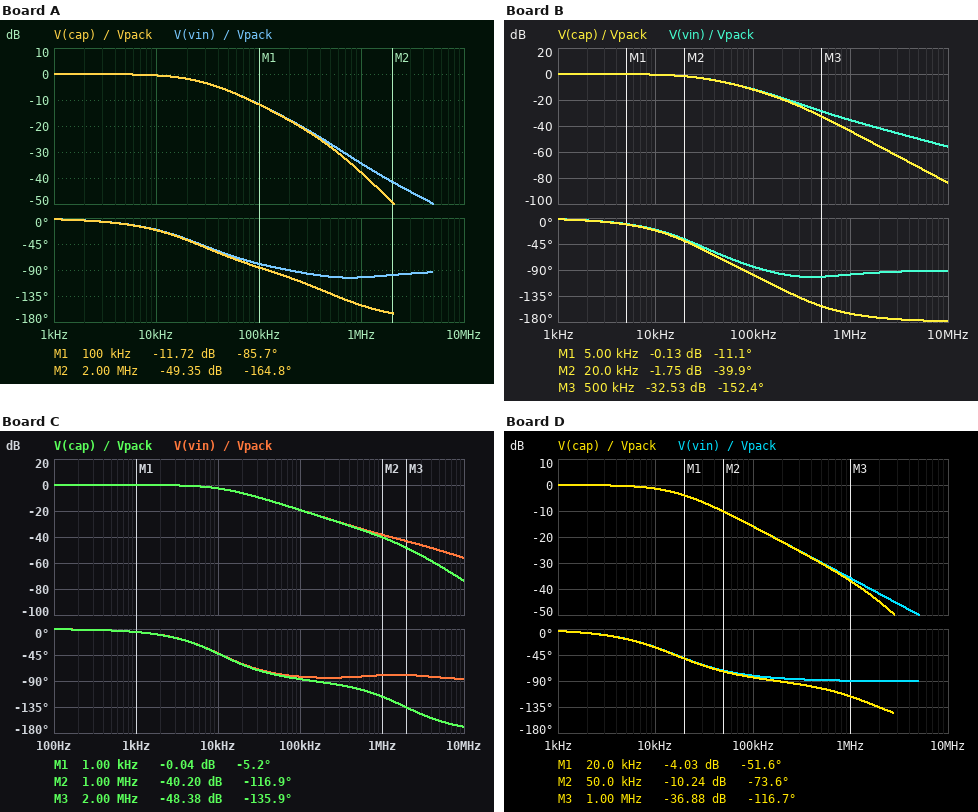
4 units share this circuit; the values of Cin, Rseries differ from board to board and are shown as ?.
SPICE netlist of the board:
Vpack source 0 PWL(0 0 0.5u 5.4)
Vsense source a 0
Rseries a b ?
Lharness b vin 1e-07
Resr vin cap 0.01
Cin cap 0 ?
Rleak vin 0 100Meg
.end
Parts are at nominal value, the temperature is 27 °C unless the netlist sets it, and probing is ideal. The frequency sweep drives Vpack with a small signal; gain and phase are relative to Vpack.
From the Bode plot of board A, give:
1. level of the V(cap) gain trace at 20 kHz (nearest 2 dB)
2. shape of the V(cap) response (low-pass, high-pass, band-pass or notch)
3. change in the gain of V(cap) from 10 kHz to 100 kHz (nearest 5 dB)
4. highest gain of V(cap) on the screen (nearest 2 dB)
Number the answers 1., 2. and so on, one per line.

1. -2 dB
2. low-pass
3. -10 dB
4. 0 dB
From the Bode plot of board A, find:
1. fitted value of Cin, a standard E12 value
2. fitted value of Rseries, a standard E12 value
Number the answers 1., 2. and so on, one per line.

1. 18 µF
2. 0.33 Ω
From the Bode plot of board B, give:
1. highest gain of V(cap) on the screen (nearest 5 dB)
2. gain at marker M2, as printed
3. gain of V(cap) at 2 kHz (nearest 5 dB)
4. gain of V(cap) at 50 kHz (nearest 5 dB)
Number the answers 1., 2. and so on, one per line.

1. 0 dB
2. -1.75 dB
3. 0 dB
4. -5 dB
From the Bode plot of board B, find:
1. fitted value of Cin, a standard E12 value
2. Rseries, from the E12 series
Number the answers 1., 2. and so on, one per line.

1. 39 µF
2. 0.15 Ω
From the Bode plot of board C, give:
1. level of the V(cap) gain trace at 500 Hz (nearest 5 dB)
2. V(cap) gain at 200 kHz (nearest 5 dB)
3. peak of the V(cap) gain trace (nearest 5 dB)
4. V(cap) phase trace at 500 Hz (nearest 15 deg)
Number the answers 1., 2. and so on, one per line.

1. 0 dB
2. -25 dB
3. 0 dB
4. 0 deg
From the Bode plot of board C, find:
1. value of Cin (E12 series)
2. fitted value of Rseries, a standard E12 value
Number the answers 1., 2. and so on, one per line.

1. 12 µF
2. 1.2 Ω
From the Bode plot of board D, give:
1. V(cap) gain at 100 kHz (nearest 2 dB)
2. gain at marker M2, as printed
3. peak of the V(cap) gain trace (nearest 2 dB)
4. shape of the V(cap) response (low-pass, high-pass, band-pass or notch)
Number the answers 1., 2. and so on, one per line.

1. -16 dB
2. -10.24 dB
3. 0 dB
4. low-pass
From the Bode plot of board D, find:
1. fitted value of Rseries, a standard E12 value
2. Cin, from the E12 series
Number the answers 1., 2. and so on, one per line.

1. 1.2 Ω
2. 8.2 µF
